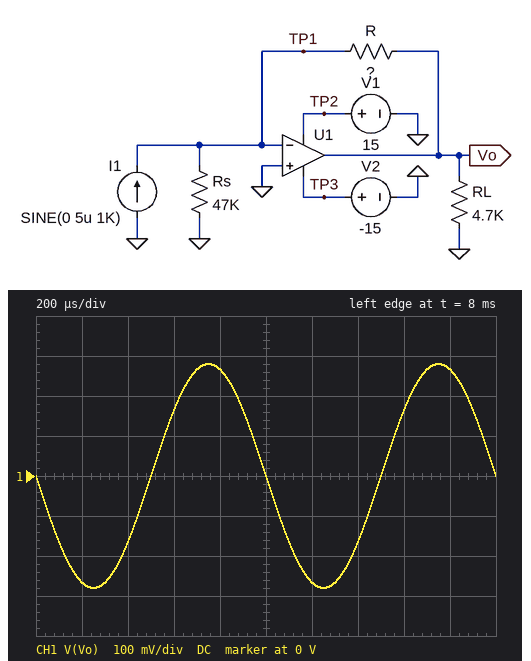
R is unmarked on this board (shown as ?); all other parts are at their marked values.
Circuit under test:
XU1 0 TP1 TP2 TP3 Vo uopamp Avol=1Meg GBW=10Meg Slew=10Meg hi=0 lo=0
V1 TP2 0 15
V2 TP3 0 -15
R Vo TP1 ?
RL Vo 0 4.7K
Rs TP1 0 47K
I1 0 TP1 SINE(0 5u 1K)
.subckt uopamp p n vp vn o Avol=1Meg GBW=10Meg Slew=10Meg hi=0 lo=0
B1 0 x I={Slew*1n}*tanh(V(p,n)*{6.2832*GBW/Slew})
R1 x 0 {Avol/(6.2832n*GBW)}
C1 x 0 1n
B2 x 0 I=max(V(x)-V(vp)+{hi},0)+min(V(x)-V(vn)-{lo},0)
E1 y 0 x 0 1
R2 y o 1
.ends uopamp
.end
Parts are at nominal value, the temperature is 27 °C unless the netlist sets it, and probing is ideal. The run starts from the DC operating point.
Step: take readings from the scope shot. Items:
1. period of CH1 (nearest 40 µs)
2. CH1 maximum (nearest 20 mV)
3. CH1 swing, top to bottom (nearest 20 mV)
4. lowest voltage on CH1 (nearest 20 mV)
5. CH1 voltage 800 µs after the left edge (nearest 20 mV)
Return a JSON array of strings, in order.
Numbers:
["1.00 ms", "280 mV", "560 mV", "-280 mV", "260 mV"]
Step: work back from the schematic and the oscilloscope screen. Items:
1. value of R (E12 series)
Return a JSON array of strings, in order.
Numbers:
["56 kΩ"]
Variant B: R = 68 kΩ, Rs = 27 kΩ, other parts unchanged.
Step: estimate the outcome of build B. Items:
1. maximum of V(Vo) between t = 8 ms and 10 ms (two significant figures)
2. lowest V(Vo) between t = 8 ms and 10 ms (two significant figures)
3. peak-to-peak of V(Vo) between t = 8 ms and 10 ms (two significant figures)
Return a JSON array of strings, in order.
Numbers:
["340 mV", "-340 mV", "680 mV"]
